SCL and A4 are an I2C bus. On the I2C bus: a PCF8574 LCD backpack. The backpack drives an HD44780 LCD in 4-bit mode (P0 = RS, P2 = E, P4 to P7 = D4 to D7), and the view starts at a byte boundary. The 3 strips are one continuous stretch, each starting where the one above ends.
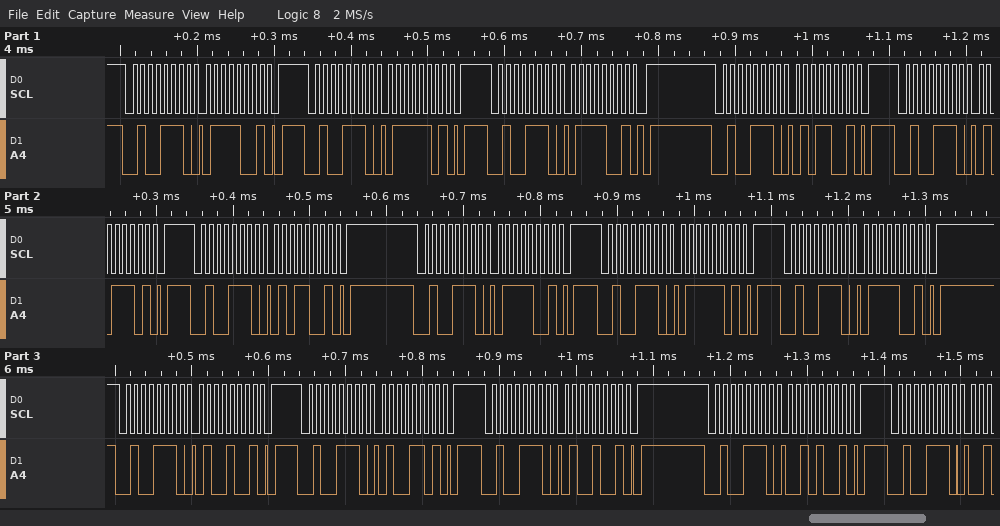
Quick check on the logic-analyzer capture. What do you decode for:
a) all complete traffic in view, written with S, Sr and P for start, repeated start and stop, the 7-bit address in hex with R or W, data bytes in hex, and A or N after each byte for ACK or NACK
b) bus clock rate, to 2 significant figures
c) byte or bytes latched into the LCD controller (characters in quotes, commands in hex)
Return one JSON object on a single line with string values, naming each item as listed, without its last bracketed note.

{"all complete traffic in view, written with S, Sr and P for start, repeated start and stop, the 7-bit address in hex with R or W, data bytes in hex, and A or N after each byte for ACK or NACK": "S 27W A 79 A P S 27W A 7D A P S 27W A 79 A P S 27W A 59 A P S 27W A 5D A P S 27W A 59 A P S 27W A 79 A P S 27W A 7D A P S 27W A 79 A P S 27W A 49 A P S 27W A 4D A P S 27W A 49 A P S 27W A 29 A P S 27W A", "bus clock rate, to 2 significant figures": "100 kHz", "byte or bytes latched into the LCD controller": "'u' 't'"}
